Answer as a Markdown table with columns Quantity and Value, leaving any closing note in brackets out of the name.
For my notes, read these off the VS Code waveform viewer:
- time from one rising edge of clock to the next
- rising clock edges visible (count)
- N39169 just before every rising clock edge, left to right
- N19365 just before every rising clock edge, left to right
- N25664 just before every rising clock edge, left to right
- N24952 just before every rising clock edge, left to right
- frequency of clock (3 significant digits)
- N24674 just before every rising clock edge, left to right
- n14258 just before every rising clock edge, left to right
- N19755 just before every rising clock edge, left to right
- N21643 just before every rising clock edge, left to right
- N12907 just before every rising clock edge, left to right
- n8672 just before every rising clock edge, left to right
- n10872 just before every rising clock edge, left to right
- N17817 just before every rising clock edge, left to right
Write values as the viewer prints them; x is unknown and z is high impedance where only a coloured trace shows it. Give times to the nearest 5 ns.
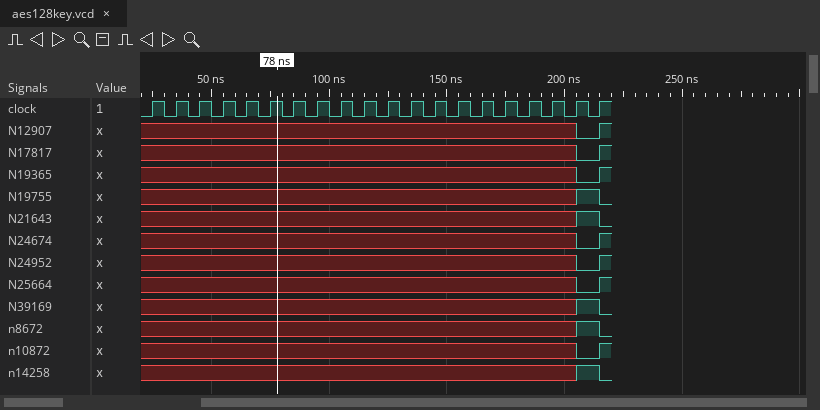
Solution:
| Quantity | Value |
|---|---|
| time from one rising edge of clock to the next | 10 ns |
| rising clock edges visible | 20 |
| N39169 just before every rising clock edge, left to right | x x x x x x x x x x x x x x x x x x x 1 |
| N19365 just before every rising clock edge, left to right | x x x x x x x x x x x x x x x x x x x 0 |
| N25664 just before every rising clock edge, left to right | x x x x x x x x x x x x x x x x x x x 0 |
| N24952 just before every rising clock edge, left to right | x x x x x x x x x x x x x x x x x x x 0 |
| frequency of clock | 100 MHz |
| N24674 just before every rising clock edge, left to right | x x x x x x x x x x x x x x x x x x x 0 |
| n14258 just before every rising clock edge, left to right | x x x x x x x x x x x x x x x x x x x 1 |
| N19755 just before every rising clock edge, left to right | x x x x x x x x x x x x x x x x x x x 1 |
| N21643 just before every rising clock edge, left to right | x x x x x x x x x x x x x x x x x x x 1 |
| N12907 just before every rising clock edge, left to right | x x x x x x x x x x x x x x x x x x x 0 |
| n8672 just before every rising clock edge, left to right | x x x x x x x x x x x x x x x x x x x 1 |
| n10872 just before every rising clock edge, left to right | x x x x x x x x x x x x x x x x x x x 0 |
| N17817 just before every rising clock edge, left to right | x x x x x x x x x x x x x x x x x x x 0 |
